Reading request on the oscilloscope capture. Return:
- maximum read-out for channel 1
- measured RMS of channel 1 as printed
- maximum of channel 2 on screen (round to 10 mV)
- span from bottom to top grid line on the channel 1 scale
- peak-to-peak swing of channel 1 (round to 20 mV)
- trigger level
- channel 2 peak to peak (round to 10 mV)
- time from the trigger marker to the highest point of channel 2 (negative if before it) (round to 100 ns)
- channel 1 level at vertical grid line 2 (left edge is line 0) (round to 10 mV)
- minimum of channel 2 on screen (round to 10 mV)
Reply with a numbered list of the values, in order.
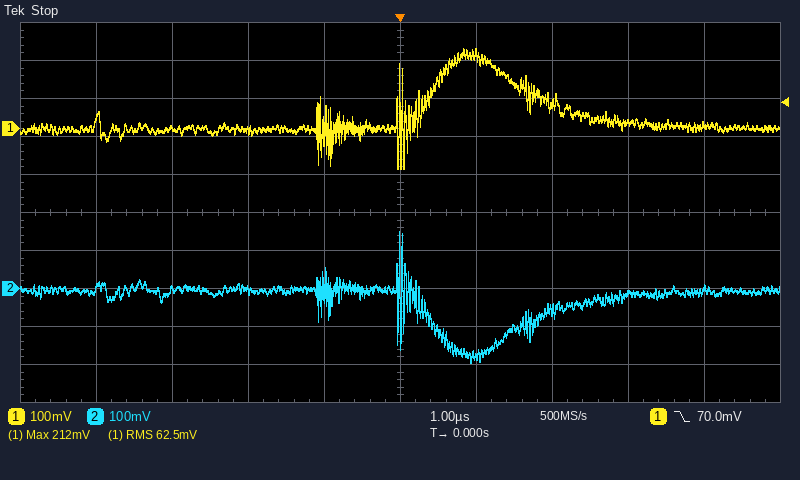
1. 212 mV
2. 62.5 mV
3. 150 mV
4. 1 V
5. 320 mV
6. 70.0 mV
7. 340 mV
8. 0.0 µs
9. 0 mV
10. -190 mV
